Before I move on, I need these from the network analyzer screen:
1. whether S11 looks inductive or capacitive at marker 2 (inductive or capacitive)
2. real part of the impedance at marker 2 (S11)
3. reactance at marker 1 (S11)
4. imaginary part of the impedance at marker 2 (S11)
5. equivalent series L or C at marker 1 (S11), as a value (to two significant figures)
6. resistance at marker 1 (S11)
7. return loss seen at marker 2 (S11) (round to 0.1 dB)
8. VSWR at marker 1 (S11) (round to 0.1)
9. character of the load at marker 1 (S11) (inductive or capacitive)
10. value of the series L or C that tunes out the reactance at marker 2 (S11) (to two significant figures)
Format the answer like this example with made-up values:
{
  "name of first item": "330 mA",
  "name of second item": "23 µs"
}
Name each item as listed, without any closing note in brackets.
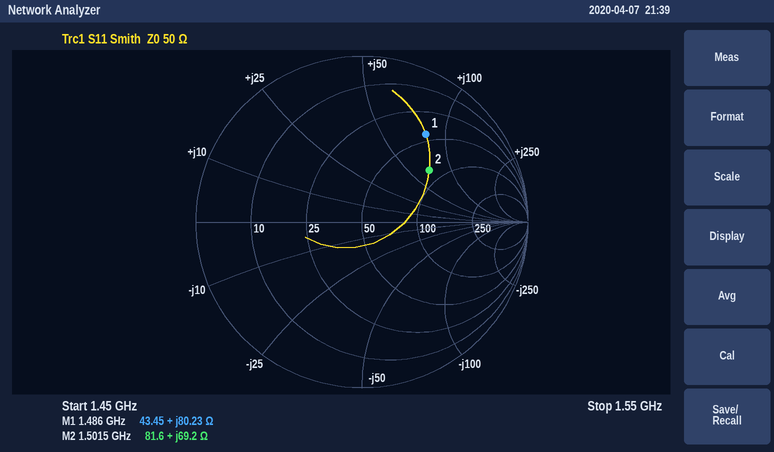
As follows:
{
  "whether S11 looks inductive or capacitive at marker 2": "inductive",
  "real part of the impedance at marker 2": "81.6 Ω",
  "reactance at marker 1": "+80.23 Ω",
  "imaginary part of the impedance at marker 2": "+69.2 Ω",
  "equivalent series L or C at marker 1 (S11), as a value": "8.6 nH",
  "resistance at marker 1": "43.45 Ω",
  "return loss seen at marker 2 (S11)": "5.8 dB",
  "VSWR at marker 1 (S11)": "4.8",
  "character of the load at marker 1 (S11)": "inductive",
  "value of the series L or C that tunes out the reactance at marker 2 (S11)": "1.5 pF"
}
